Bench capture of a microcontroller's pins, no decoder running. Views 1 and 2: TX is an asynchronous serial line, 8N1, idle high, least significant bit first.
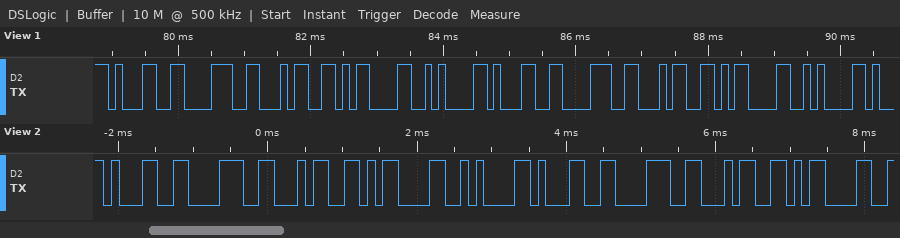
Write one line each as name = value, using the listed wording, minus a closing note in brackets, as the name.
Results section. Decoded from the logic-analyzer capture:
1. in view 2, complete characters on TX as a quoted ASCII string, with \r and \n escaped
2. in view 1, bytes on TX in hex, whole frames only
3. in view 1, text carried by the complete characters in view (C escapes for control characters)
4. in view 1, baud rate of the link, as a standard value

in view 2, complete characters on TX as a quoted ASCII string, with \r and \n escaped = "184\r\n184\r"
in view 1, bytes on TX in hex, whole frames only = 31 38 34 0D 0A 31 38 34 0D 0A
in view 1, text carried by the complete characters in view = "184\r\n184\r\n"
in view 1, baud rate of the link, as a standard value = 9600 baud
